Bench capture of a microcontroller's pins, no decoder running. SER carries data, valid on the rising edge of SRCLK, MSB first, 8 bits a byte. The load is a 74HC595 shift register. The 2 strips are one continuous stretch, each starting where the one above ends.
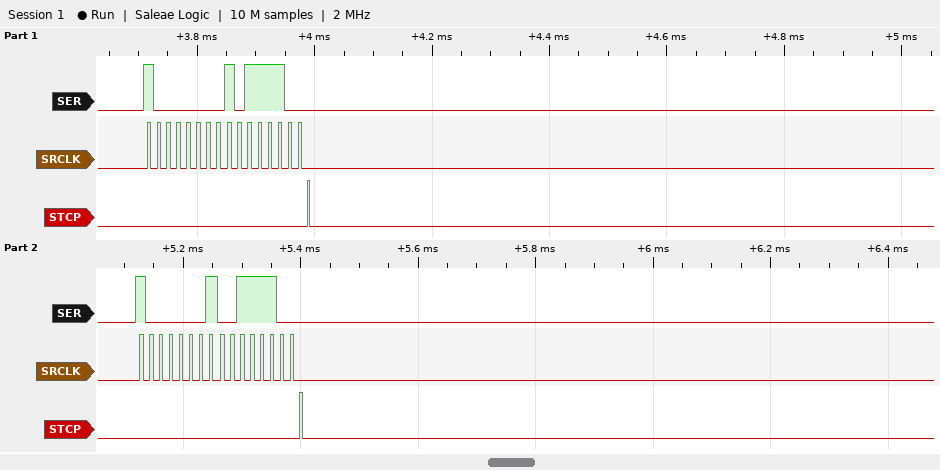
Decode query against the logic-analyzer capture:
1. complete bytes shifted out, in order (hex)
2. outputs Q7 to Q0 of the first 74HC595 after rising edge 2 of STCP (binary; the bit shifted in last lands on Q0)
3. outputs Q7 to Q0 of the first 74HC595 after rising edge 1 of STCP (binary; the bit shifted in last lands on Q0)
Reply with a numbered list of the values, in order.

1. 0x80 0xBC 0x81 0x3C
2. 00111100
3. 10111100
